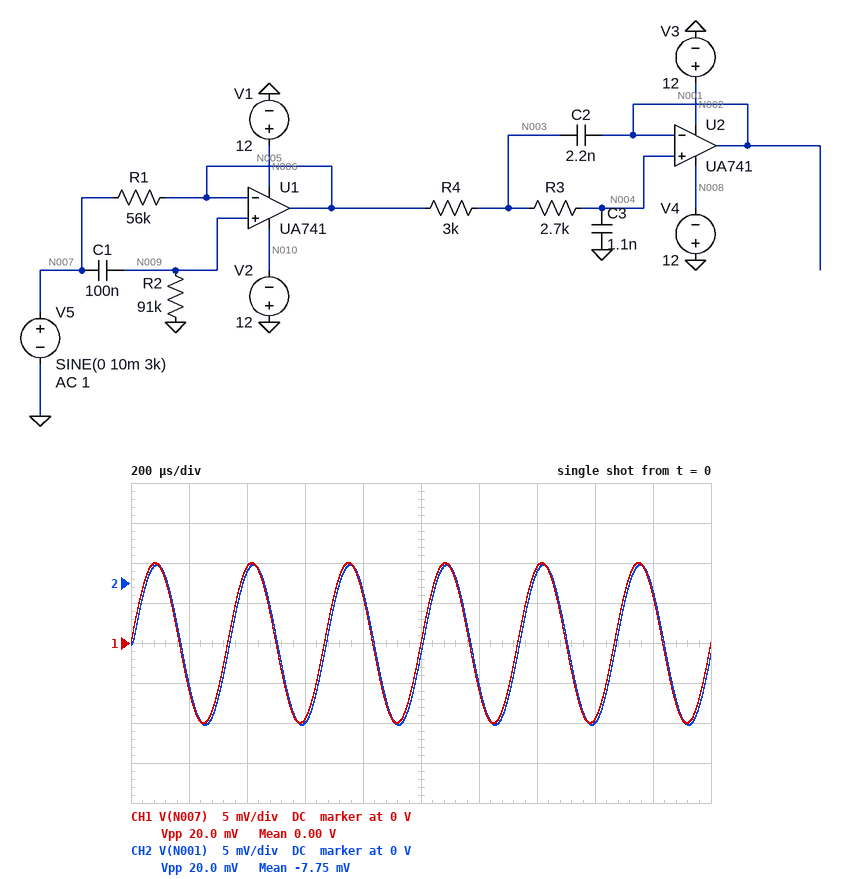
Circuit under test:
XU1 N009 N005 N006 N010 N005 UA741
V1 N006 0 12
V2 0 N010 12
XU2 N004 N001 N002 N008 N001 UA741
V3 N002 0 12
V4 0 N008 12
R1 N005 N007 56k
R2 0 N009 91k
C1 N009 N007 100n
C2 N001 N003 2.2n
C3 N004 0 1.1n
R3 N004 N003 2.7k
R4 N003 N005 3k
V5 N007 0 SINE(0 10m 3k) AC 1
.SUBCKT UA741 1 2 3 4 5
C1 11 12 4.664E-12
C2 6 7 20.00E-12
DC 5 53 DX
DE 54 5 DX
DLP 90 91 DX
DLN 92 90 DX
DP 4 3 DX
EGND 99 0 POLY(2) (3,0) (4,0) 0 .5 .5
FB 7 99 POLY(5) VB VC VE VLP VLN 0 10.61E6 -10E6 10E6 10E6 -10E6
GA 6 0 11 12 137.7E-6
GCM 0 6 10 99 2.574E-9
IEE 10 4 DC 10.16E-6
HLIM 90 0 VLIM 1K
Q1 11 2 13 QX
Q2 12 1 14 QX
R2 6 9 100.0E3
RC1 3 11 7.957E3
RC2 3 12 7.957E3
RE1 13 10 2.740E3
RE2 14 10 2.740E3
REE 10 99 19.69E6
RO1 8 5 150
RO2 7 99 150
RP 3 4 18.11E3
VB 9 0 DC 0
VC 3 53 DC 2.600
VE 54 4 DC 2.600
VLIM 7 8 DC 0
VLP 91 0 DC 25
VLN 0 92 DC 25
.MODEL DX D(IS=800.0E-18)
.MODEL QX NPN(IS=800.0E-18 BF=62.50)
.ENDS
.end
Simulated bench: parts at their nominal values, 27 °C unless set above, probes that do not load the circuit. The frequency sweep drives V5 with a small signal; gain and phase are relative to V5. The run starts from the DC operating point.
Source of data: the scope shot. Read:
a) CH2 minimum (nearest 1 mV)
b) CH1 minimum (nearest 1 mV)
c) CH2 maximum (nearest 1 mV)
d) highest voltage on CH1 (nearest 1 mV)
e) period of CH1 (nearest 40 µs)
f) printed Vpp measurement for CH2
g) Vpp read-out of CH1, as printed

-18 mV
-10 mV
2 mV
10 mV
320 µs
20.0 mV
20.0 mV
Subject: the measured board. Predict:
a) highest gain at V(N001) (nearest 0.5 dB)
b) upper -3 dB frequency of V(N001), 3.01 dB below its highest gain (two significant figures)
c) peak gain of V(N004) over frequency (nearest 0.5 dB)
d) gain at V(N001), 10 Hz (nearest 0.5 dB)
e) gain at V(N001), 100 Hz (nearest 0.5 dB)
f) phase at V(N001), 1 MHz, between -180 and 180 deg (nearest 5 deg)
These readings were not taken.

0 dB
36 kHz
0 dB
-6.0 dB
0 dB
-5 deg
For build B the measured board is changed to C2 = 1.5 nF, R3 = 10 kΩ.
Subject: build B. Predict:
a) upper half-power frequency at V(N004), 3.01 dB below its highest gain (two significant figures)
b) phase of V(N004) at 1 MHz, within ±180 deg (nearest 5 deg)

14 kHz
-140 deg
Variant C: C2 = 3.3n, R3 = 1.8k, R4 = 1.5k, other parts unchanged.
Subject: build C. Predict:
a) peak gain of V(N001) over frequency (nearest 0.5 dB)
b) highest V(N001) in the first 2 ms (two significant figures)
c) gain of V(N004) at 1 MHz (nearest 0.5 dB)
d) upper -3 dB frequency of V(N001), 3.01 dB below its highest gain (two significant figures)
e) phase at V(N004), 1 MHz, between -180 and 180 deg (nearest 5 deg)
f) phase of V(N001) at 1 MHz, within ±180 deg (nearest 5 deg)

0.5 dB
2.5 mV
-47.5 dB
56 kHz
-110 deg
-10 deg
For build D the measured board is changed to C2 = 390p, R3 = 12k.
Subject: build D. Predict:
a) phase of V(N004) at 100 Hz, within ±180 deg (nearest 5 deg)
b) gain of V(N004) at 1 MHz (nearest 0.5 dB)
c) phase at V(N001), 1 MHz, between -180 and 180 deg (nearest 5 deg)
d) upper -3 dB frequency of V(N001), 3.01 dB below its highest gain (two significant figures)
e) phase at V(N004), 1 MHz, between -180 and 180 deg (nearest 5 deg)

10 deg
-59.5 dB
5 deg
10 kHz
140 deg
